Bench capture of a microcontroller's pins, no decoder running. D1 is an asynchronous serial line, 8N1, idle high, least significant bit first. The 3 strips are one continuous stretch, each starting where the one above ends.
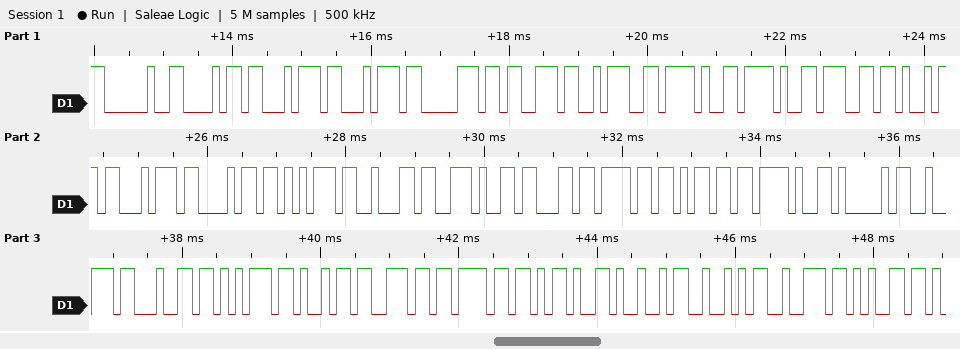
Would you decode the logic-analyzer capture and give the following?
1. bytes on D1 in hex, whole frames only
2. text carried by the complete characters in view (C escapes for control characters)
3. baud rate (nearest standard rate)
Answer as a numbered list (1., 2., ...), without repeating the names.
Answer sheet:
1. 20 68 74 74 70 73 3A 2F 2F 67 69 74 68 75 62 2E 63 6F 6D 2F 41 72 64 75 69 6E 6F 2D 49 52 72 65
2. " https://github.com/Arduino-IRre"
3. 9600 baud
